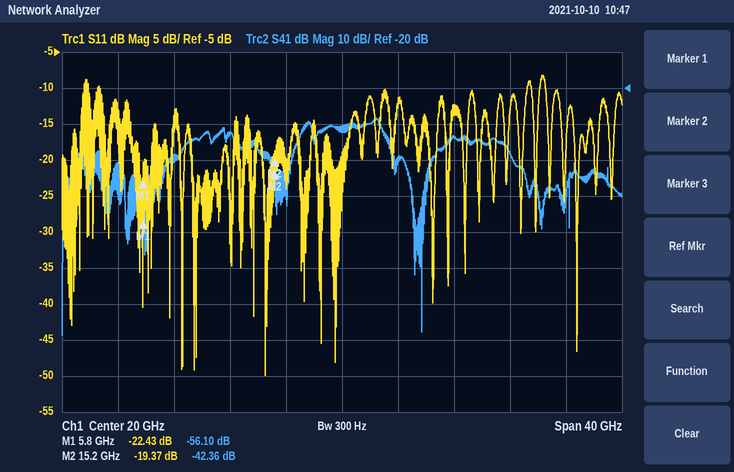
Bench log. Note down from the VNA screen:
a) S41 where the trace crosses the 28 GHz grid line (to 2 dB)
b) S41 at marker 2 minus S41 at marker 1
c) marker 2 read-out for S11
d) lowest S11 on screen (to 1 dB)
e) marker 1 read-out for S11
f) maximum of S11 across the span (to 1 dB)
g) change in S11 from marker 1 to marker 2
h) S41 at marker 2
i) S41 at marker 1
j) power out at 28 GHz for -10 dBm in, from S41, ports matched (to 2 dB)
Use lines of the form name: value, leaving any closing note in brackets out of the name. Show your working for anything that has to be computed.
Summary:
S41 where the trace crosses the 28 GHz grid line: -34 dB
S41 at marker 2 minus S41 at marker 1: -42.36 − (-56.1) = 13.74 dB
marker 2 read-out for S11: -19.37 dB
lowest S11 on screen: -50 dB
marker 1 read-out for S11: -22.43 dB
maximum of S11 across the span: -8 dB
change in S11 from marker 1 to marker 2: -19.37 − (-22.43) = 3.06 dB
S41 at marker 2: -42.36 dB
S41 at marker 1: -56.10 dB
power out at 28 GHz for -10 dBm in, from S41, ports matched: -10 dBm + (-34 dB) = -44 dBm
